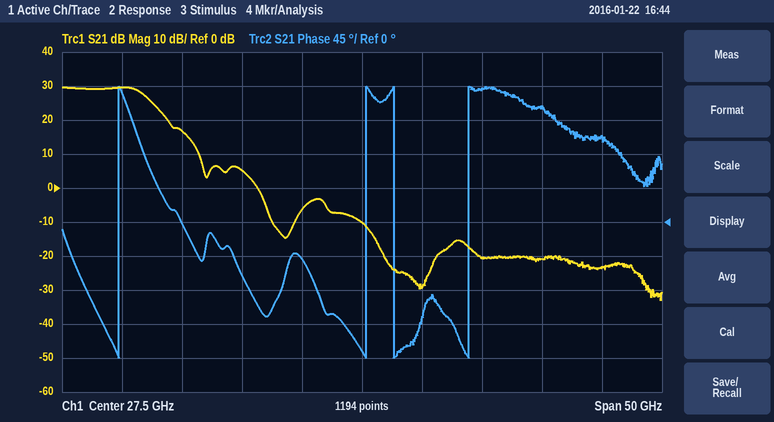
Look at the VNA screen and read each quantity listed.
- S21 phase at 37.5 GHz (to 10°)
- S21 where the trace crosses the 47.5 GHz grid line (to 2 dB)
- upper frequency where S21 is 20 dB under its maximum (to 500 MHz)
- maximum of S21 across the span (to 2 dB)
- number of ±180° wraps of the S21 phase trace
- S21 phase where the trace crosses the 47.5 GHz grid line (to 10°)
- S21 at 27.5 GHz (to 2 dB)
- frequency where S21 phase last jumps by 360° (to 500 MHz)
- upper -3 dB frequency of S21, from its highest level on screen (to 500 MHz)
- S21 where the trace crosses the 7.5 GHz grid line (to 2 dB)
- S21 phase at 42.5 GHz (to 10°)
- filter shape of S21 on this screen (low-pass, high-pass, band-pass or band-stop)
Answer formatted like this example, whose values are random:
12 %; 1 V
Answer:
180°; -24 dB; 14.0 GHz; 30 dB; 4; 110°; -10 dB; 36.5 GHz; 9.5 GHz; 30 dB; 150°; low-pass
